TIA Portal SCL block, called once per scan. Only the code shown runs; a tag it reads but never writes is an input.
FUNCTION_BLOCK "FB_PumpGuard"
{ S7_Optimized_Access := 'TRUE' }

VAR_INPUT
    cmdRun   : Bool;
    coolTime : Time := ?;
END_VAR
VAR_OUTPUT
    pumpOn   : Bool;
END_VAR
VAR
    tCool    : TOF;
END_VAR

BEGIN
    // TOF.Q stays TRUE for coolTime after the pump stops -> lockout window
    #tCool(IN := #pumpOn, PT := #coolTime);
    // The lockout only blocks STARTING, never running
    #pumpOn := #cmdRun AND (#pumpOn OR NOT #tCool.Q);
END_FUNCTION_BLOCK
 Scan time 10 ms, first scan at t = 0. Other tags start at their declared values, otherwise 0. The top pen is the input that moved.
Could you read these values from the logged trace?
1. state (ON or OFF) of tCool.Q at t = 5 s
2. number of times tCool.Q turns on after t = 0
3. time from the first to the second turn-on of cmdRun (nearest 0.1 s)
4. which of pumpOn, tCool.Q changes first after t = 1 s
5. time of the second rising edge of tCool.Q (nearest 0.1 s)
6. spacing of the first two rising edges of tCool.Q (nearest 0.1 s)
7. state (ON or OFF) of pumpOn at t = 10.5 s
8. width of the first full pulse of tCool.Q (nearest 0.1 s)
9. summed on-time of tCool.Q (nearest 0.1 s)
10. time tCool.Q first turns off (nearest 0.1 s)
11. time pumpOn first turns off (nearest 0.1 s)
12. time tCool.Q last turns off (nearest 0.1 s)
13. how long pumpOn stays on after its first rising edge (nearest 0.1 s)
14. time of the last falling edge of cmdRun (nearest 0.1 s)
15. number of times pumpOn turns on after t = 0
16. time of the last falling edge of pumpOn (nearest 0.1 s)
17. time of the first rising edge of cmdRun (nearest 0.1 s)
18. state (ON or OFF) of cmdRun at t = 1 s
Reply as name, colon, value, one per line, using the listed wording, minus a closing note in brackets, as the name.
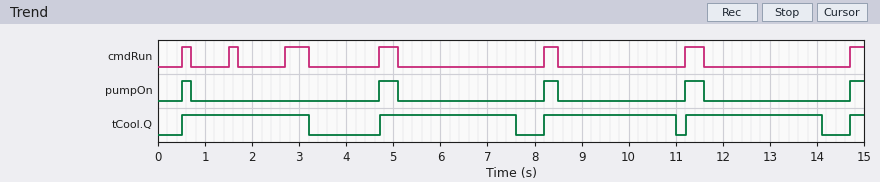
state (ON or OFF) of tCool.Q at t = 5 s: ON
number of times tCool.Q turns on after t = 0: 5
time from the first to the second turn-on of cmdRun: 1.0 s
which of pumpOn, tCool.Q changes first after t = 1 s: tCool.Q
time of the second rising edge of tCool.Q: 4.7 s
spacing of the first two rising edges of tCool.Q: 4.2 s
state (ON or OFF) of pumpOn at t = 10.5 s: OFF
width of the first full pulse of tCool.Q: 2.7 s
summed on-time of tCool.Q: 11.6 s
time tCool.Q first turns off: 3.2 s
time pumpOn first turns off: 0.7 s
time tCool.Q last turns off: 14.1 s
how long pumpOn stays on after its first rising edge: 0.2 s
time of the last falling edge of cmdRun: 11.6 s
number of times pumpOn turns on after t = 0: 5
time of the last falling edge of pumpOn: 11.6 s
time of the first rising edge of cmdRun: 0.5 s
state (ON or OFF) of cmdRun at t = 1 s: OFF
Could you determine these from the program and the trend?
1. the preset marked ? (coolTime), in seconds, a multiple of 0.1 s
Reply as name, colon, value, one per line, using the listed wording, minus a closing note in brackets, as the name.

the preset marked ? (coolTime), in seconds, a multiple of 0.1 s: 2.5 s
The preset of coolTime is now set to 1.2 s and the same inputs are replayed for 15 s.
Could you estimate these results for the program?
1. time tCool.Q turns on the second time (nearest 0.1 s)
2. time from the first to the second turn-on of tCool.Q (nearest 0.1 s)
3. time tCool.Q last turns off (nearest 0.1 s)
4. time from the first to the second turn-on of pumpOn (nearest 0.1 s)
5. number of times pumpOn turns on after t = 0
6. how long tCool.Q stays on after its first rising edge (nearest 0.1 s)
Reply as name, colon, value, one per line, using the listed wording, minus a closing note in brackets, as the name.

time tCool.Q turns on the second time: 2.7 s
time from the first to the second turn-on of tCool.Q: 2.2 s
time tCool.Q last turns off: 12.8 s
time from the first to the second turn-on of pumpOn: 2.2 s
number of times pumpOn turns on after t = 0: 6
how long tCool.Q stays on after its first rising edge: 1.4 s
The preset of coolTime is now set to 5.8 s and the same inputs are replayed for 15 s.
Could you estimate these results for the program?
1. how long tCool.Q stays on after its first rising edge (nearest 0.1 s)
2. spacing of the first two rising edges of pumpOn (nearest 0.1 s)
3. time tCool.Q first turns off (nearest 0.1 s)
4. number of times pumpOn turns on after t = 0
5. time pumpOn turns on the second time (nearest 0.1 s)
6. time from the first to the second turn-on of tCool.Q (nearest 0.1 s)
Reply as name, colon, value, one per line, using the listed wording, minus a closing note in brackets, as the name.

how long tCool.Q stays on after its first rising edge: 6.0 s
spacing of the first two rising edges of pumpOn: 7.7 s
time tCool.Q first turns off: 6.5 s
number of times pumpOn turns on after t = 0: 3
time pumpOn turns on the second time: 8.2 s
time from the first to the second turn-on of tCool.Q: 7.7 s
